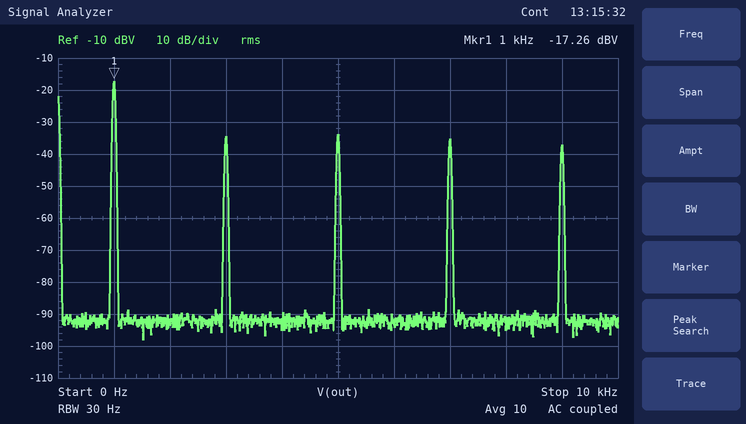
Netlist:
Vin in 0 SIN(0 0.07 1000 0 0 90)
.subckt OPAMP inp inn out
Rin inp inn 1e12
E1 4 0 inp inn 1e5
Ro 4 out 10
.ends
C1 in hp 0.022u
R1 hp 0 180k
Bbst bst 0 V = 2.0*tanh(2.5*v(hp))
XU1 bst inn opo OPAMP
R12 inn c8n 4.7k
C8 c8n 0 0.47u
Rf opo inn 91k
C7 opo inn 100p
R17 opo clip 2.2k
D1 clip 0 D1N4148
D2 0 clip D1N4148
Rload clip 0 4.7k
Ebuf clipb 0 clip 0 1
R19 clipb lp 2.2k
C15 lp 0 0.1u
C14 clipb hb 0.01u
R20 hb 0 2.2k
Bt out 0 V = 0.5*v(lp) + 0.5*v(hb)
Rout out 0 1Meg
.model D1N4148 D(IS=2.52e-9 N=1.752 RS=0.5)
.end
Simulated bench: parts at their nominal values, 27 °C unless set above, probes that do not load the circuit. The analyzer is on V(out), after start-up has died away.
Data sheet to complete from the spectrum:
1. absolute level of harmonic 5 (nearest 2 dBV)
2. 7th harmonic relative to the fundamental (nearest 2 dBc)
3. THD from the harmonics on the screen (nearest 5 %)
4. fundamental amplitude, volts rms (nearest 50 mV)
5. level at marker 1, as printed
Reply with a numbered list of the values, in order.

1. -34 dBV
2. -18 dBc
3. 25 %
4. 150 mV
5. -17.26 dBV
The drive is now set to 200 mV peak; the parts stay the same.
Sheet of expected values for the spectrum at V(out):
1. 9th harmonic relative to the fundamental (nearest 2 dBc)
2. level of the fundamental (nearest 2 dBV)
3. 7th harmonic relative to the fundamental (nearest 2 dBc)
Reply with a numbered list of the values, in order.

1. -18 dBc
2. -16 dBV
3. -16 dBc
